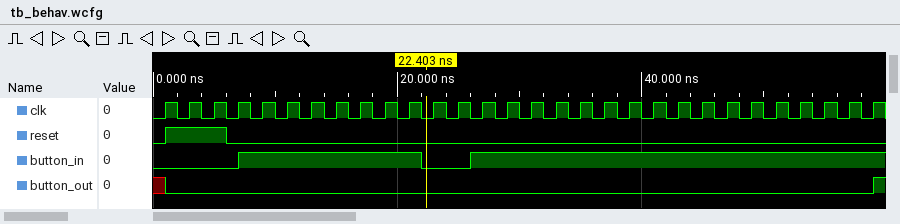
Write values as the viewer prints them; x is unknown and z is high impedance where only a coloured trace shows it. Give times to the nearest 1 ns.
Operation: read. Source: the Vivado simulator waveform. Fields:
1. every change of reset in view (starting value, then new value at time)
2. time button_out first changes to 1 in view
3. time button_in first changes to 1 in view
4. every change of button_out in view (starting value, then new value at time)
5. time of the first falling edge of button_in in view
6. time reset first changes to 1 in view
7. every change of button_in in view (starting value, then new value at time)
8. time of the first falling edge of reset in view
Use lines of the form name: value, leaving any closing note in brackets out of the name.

every change of reset in view: 0, 1 at 1 ns, 0 at 6 ns
time button_out first changes to 1 in view: 59 ns
time button_in first changes to 1 in view: 7 ns
every change of button_out in view: x, 0 at 1 ns, 1 at 59 ns
time of the first falling edge of button_in in view: 22 ns
time reset first changes to 1 in view: 1 ns
every change of button_in in view: 0, 1 at 7 ns, 0 at 22 ns, 1 at 26 ns
time of the first falling edge of reset in view: 6 ns
